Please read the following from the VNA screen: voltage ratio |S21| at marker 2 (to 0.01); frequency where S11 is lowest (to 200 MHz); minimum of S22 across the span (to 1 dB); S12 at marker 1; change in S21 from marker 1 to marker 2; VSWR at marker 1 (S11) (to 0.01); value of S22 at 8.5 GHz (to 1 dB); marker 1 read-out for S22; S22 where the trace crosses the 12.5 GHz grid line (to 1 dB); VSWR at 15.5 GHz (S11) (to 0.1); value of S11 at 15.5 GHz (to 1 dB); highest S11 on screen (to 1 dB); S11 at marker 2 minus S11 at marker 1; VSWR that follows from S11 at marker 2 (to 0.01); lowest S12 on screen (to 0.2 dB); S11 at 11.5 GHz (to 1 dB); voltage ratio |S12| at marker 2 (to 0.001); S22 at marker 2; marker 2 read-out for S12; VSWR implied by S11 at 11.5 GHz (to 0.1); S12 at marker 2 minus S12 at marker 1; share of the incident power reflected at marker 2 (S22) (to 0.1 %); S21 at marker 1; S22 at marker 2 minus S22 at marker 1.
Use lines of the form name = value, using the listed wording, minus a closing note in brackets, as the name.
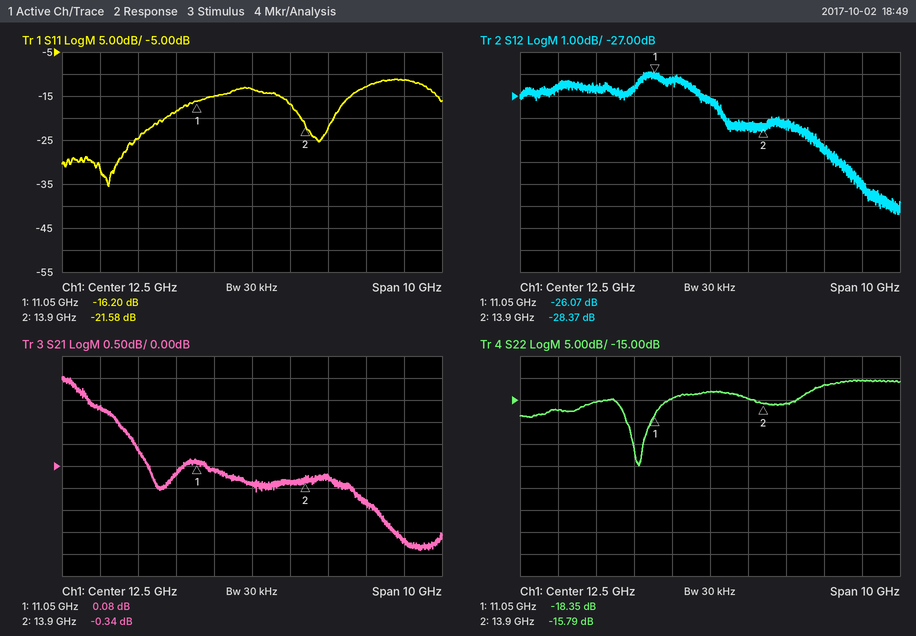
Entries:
voltage ratio |S21| at marker 2 = 0.96
frequency where S11 is lowest = 8.8 GHz
minimum of S22 across the span = -30 dB
S12 at marker 1 = -26.07 dB
change in S21 from marker 1 to marker 2 = -0.42 dB
VSWR at marker 1 (S11) = 1.37
value of S22 at 8.5 GHz = -17 dB
marker 1 read-out for S22 = -18.35 dB
S22 where the trace crosses the 12.5 GHz grid line = -13 dB
VSWR at 15.5 GHz (S11) = 1.6
value of S11 at 15.5 GHz = -13 dB
highest S11 on screen = -11 dB
S11 at marker 2 minus S11 at marker 1 = -5.38 dB
VSWR that follows from S11 at marker 2 = 1.18
lowest S12 on screen = -32.4 dB
S11 at 11.5 GHz = -15 dB
voltage ratio |S12| at marker 2 = 0.038
S22 at marker 2 = -15.79 dB
marker 2 read-out for S12 = -28.37 dB
VSWR implied by S11 at 11.5 GHz = 1.4
S12 at marker 2 minus S12 at marker 1 = -2.30 dB
share of the incident power reflected at marker 2 (S22) = 2.6 %
S21 at marker 1 = 0.08 dB
S22 at marker 2 minus S22 at marker 1 = 2.56 dB
